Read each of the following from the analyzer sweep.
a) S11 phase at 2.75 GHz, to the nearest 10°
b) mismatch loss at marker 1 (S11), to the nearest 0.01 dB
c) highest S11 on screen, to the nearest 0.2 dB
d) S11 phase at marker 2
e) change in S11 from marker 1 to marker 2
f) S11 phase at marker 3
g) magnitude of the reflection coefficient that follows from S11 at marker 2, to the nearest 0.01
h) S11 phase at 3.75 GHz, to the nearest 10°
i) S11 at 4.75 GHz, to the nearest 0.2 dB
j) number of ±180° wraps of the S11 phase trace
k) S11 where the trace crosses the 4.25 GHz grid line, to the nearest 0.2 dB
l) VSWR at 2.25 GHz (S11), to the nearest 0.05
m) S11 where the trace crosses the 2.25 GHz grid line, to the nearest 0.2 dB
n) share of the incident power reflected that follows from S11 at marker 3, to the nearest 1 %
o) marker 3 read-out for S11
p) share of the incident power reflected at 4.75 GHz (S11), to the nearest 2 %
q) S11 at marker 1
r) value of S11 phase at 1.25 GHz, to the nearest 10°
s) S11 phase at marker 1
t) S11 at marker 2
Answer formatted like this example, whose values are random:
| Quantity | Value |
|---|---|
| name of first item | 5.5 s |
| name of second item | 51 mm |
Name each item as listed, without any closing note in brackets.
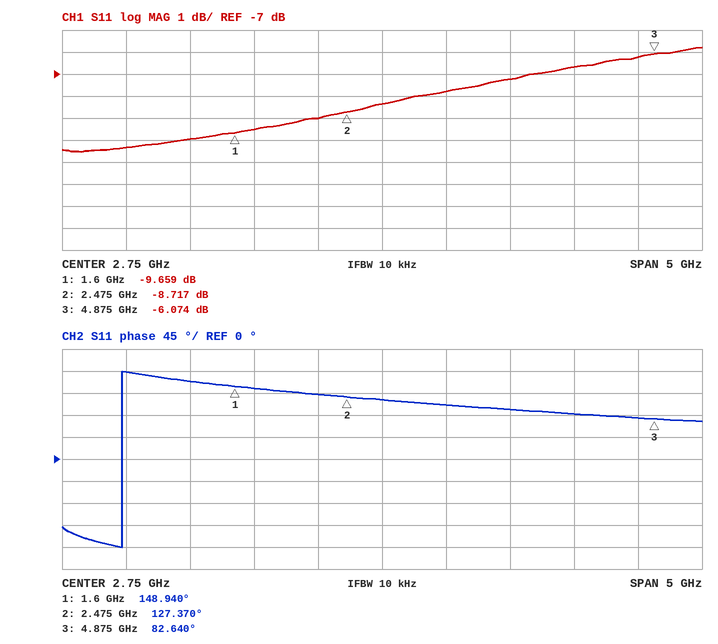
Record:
| Quantity | Value |
|---|---|
| S11 phase at 2.75 GHz, to the nearest 10° | 120° |
| mismatch loss at marker 1 (S11), to the nearest 0.01 dB | 0.50 dB |
| highest S11 on screen, to the nearest 0.2 dB | -5.8 dB |
| S11 phase at marker 2 | 127.370° |
| change in S11 from marker 1 to marker 2 | 0.942 dB |
| S11 phase at marker 3 | 82.640° |
| magnitude of the reflection coefficient that follows from S11 at marker 2, to the nearest 0.01 | 0.37 |
| S11 phase at 3.75 GHz, to the nearest 10° | 100° |
| S11 at 4.75 GHz, to the nearest 0.2 dB | -6.2 dB |
| number of ±180° wraps of the S11 phase trace | 1 |
| S11 where the trace crosses the 4.25 GHz grid line, to the nearest 0.2 dB | -6.6 dB |
| VSWR at 2.25 GHz (S11), to the nearest 0.05 | 2.10 |
| S11 where the trace crosses the 2.25 GHz grid line, to the nearest 0.2 dB | -9.0 dB |
| share of the incident power reflected that follows from S11 at marker 3, to the nearest 1 % | 25 % |
| marker 3 read-out for S11 | -6.074 dB |
| share of the incident power reflected at 4.75 GHz (S11), to the nearest 2 % | 24 % |
| S11 at marker 1 | -9.659 dB |
| value of S11 phase at 1.25 GHz, to the nearest 10° | 160° |
| S11 phase at marker 1 | 148.940° |
| S11 at marker 2 | -8.717 dB |
